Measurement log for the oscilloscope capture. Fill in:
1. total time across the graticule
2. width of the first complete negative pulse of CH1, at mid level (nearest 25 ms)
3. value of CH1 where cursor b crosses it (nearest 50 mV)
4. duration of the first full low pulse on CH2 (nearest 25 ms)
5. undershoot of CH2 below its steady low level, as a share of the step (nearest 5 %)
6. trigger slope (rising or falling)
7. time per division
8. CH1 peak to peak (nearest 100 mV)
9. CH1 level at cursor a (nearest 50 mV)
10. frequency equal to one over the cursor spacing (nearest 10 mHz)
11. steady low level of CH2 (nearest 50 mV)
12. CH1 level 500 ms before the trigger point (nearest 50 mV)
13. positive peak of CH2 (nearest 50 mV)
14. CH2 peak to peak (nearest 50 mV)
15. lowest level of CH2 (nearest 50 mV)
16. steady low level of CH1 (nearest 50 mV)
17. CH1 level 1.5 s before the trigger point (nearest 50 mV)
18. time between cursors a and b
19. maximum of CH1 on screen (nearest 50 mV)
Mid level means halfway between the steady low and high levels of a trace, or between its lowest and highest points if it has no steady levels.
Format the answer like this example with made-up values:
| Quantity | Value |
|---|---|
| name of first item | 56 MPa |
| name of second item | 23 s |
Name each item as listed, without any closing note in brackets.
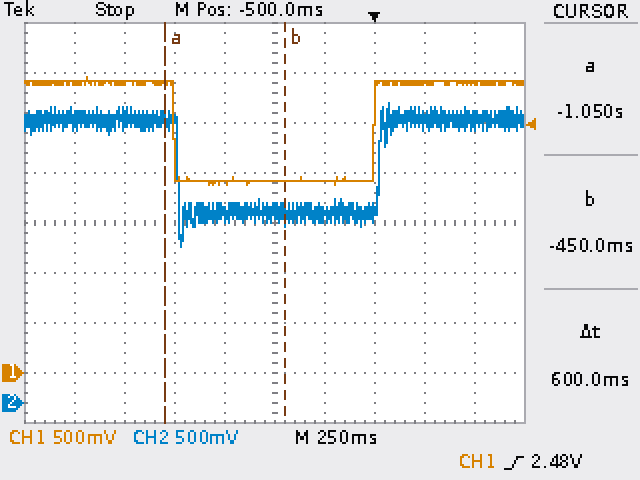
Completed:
| Quantity | Value |
|---|---|
| total time across the graticule | 2.5 s |
| width of the first complete negative pulse of CH1, at mid level | 1.000 s |
| value of CH1 where cursor b crosses it | 1.90 V |
| duration of the first full low pulse on CH2 | 1.000 s |
| undershoot of CH2 below its steady low level, as a share of the step | 35 % |
| trigger slope | rising |
| time per division | 250 ms |
| CH1 peak to peak | 1.10 V |
| CH1 level at cursor a | 2.90 V |
| frequency equal to one over the cursor spacing | 1.67 Hz |
| steady low level of CH2 | 1.90 V |
| CH1 level 500 ms before the trigger point | 1.90 V |
| positive peak of CH2 | 3.00 V |
| CH2 peak to peak | 1.45 V |
| lowest level of CH2 | 1.55 V |
| steady low level of CH1 | 1.90 V |
| CH1 level 1.5 s before the trigger point | 2.90 V |
| time between cursors a and b | 600 ms |
| maximum of CH1 on screen | 2.95 V |
